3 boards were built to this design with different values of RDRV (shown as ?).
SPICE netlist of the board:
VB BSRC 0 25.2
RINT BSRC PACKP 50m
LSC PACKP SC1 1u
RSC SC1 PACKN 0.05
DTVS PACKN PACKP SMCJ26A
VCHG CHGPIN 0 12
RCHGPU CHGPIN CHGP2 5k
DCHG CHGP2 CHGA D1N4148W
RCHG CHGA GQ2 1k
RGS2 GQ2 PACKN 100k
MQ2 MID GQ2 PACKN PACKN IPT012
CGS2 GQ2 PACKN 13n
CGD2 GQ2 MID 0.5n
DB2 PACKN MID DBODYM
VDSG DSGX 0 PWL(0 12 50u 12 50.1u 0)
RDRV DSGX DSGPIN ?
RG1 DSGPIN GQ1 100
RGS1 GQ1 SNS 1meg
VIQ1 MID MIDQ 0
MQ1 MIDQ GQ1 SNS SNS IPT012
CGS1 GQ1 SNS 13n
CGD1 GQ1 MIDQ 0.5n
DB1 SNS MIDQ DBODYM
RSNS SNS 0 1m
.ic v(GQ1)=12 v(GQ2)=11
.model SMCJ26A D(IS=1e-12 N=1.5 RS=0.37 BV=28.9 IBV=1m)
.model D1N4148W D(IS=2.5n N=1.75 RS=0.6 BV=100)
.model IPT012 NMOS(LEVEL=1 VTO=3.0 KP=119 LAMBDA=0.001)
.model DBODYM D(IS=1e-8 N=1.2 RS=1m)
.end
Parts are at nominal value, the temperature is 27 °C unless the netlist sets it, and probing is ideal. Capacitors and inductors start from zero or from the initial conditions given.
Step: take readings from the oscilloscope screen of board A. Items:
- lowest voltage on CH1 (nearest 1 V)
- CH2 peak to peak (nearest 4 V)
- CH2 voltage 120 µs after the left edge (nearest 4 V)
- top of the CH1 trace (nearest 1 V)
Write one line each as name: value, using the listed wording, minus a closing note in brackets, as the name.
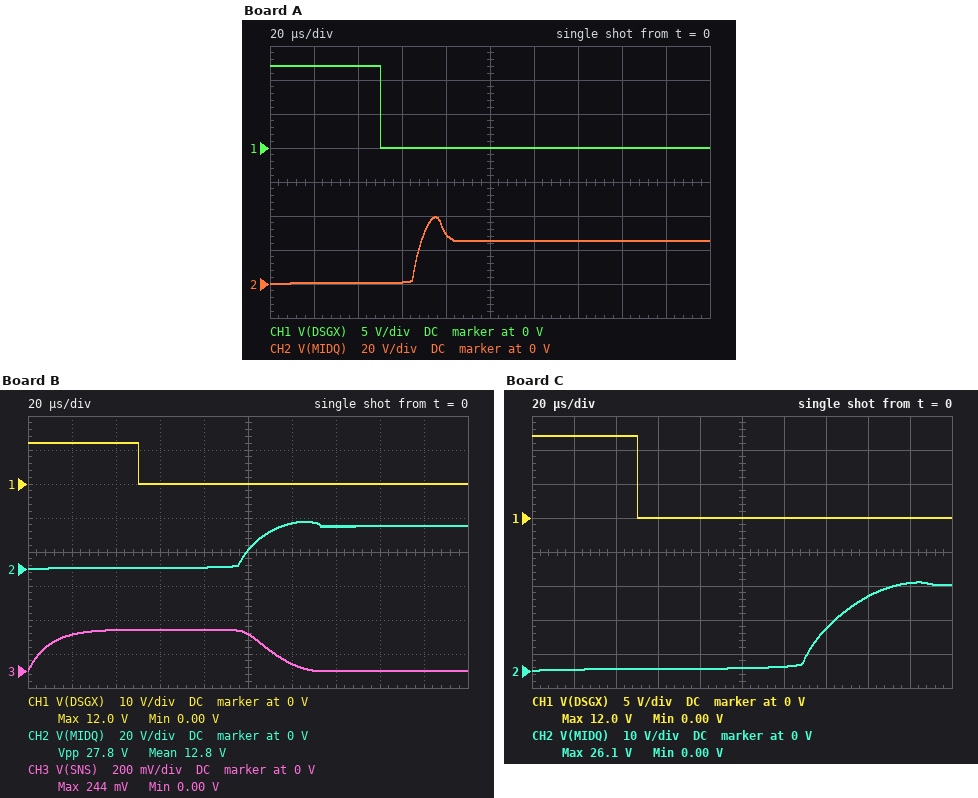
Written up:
lowest voltage on CH1: 0 V
CH2 peak to peak: 40 V
CH2 voltage 120 µs after the left edge: 24 V
top of the CH1 trace: 12 V
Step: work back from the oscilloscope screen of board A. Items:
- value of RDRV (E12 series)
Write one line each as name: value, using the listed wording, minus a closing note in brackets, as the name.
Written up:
value of RDRV: 1.2 kΩ
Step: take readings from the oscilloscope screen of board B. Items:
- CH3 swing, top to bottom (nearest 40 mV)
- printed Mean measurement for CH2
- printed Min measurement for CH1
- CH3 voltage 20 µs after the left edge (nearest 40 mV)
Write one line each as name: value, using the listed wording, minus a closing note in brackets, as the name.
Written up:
CH3 swing, top to bottom: 240 mV
printed Mean measurement for CH2: 12.8 V
printed Min measurement for CH1: 0.00 V
CH3 voltage 20 µs after the left edge: 200 mV
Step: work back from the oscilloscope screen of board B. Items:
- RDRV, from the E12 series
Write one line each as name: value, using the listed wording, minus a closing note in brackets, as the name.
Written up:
RDRV, from the E12 series: 3.9 kΩ
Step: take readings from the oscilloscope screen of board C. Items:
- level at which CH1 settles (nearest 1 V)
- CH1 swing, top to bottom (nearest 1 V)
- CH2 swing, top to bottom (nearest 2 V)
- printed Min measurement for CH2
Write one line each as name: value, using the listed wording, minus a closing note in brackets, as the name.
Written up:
level at which CH1 settles: 0 V
CH1 swing, top to bottom: 12 V
CH2 swing, top to bottom: 26 V
printed Min measurement for CH2: 0.00 V
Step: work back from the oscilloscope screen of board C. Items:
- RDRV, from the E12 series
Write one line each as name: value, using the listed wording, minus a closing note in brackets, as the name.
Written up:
RDRV, from the E12 series: 6.8 kΩ
